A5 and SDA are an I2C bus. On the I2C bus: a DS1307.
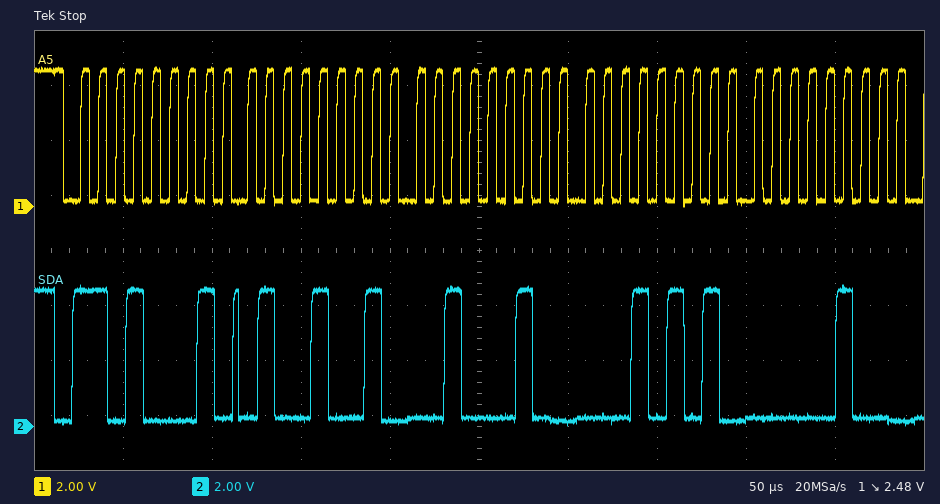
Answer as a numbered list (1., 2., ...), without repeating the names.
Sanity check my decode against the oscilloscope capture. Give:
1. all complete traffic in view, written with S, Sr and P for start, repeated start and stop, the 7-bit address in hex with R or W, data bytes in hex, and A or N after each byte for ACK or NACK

1. S 68R A 49 A 22 A 15 A 04 A
